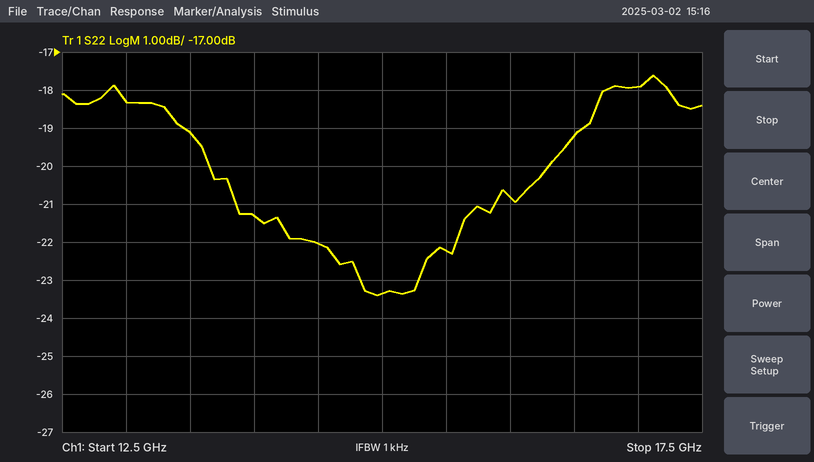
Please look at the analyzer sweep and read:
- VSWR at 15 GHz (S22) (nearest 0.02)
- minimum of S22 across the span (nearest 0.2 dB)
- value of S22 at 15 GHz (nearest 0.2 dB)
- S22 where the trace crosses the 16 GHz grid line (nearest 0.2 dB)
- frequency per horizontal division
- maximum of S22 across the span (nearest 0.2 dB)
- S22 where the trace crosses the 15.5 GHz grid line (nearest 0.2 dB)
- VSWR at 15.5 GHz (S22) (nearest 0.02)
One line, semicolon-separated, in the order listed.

1.14; -23.4 dB; -23.4 dB; -20.8 dB; 500 MHz; -17.6 dB; -22.2 dB; 1.16
